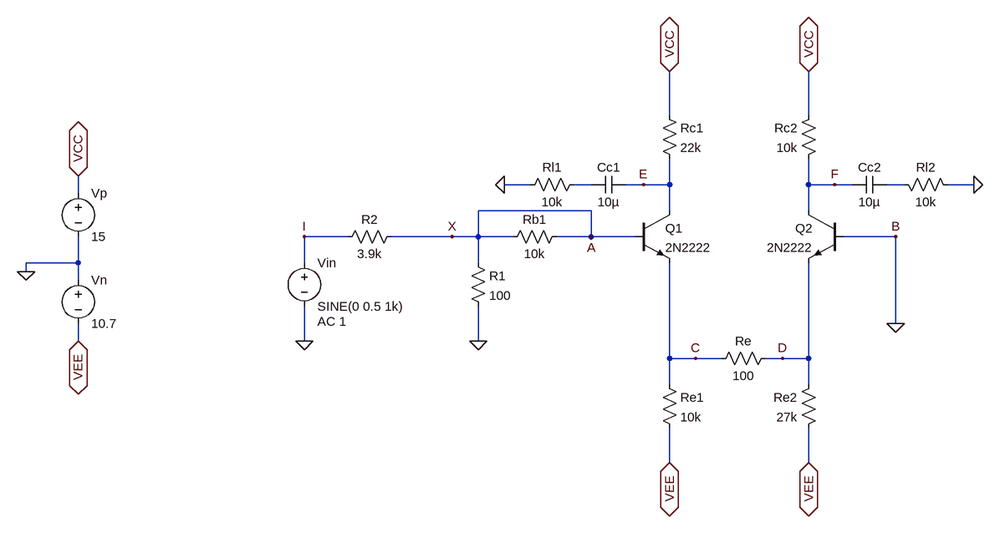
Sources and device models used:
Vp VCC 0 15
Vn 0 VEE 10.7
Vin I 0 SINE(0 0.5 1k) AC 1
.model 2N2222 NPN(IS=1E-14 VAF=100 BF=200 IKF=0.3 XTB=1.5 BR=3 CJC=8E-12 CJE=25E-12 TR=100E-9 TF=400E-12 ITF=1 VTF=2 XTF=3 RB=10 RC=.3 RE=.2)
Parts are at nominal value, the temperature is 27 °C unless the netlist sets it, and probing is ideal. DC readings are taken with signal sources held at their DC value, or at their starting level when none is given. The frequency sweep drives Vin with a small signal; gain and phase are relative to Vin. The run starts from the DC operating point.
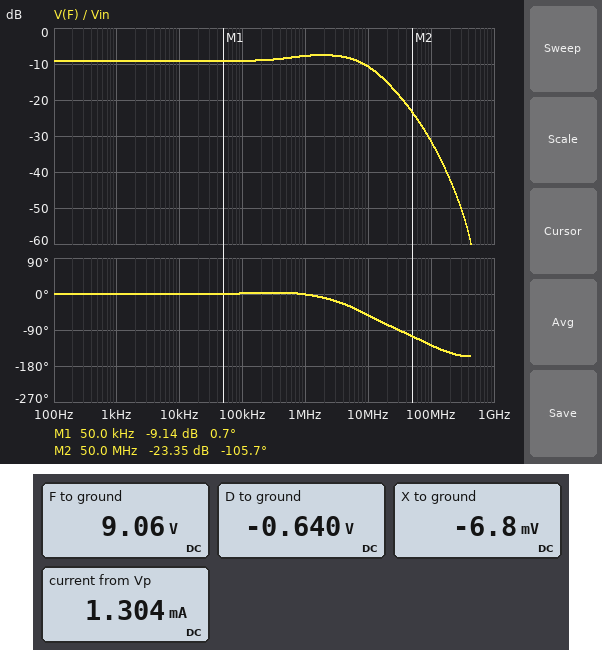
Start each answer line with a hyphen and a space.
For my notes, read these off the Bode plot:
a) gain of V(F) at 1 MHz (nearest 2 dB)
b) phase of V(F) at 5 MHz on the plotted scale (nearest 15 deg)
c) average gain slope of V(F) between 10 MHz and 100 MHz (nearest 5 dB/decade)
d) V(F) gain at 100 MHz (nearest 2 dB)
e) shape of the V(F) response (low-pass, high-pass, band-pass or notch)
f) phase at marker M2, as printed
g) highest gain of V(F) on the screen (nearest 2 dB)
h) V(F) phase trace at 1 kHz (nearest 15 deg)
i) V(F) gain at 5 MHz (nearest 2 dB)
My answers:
- -8 dB
- -30 deg
- -20 dB/decade
- -32 dB
- low-pass
- -105.7 deg
- -8 dB
- 0 deg
- -8 dB
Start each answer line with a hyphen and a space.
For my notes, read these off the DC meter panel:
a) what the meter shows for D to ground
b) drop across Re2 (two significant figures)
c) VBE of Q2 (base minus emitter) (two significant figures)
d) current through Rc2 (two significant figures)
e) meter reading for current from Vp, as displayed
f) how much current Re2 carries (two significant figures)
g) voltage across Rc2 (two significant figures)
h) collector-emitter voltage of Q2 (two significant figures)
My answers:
- -0.640 V
- 10 V
- 640 mV
- 590 µA
- 1.304 mA
- 370 µA
- 5.9 V
- 9.7 V
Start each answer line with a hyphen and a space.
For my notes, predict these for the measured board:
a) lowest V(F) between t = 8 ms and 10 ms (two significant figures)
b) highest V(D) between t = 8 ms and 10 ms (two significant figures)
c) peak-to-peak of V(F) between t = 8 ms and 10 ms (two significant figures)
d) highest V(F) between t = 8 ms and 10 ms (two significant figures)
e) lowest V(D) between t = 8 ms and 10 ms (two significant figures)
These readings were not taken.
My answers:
- 8.9 V
- -640 mV
- 350 mV
- 9.2 V
- -640 mV
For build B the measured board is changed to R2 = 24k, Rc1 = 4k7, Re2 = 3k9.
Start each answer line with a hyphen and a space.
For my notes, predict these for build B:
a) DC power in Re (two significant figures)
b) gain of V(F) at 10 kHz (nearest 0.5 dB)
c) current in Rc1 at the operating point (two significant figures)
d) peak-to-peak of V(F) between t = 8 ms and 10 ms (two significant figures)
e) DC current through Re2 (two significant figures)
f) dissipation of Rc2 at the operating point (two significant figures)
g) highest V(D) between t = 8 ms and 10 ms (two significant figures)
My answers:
- 13 µW
- -57.5 dB
- 1.4 mA
- 1.3 mV
- 2.6 mA
- 25 mW
- -700 mV
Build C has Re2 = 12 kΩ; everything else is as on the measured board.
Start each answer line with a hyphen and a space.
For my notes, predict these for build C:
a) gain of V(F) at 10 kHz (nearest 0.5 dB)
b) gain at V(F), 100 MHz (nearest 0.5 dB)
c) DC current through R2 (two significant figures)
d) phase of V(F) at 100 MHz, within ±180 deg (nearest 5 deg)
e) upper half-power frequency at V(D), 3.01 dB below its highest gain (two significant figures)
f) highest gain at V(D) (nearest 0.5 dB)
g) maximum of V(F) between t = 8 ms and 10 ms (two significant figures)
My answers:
- -8.5 dB
- -31.0 dB
- 2.9 µA
- -120 deg
- 170 MHz
- -50.0 dB
- 5.1 V
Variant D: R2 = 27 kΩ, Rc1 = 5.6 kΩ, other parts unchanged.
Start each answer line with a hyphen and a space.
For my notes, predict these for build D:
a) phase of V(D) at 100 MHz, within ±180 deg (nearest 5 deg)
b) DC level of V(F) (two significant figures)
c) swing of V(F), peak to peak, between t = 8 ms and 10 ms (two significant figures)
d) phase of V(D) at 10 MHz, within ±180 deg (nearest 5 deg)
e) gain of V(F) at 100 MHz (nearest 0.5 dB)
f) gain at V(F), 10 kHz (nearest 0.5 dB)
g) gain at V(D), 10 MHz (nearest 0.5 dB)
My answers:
- -35 deg
- 9.9 V
- 100 mV
- -15 deg
- -49.0 dB
- -20.0 dB
- -61.5 dB
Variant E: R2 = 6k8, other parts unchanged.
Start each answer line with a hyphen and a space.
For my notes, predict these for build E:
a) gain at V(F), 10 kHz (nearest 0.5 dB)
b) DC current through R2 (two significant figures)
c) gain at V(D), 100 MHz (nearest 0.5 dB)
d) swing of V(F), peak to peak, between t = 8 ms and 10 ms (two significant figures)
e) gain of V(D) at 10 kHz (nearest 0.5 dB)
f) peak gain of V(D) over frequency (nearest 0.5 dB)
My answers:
- -14.0 dB
- 1.0 µA
- -54.5 dB
- 200 mV
- -55.0 dB
- -52.0 dB
